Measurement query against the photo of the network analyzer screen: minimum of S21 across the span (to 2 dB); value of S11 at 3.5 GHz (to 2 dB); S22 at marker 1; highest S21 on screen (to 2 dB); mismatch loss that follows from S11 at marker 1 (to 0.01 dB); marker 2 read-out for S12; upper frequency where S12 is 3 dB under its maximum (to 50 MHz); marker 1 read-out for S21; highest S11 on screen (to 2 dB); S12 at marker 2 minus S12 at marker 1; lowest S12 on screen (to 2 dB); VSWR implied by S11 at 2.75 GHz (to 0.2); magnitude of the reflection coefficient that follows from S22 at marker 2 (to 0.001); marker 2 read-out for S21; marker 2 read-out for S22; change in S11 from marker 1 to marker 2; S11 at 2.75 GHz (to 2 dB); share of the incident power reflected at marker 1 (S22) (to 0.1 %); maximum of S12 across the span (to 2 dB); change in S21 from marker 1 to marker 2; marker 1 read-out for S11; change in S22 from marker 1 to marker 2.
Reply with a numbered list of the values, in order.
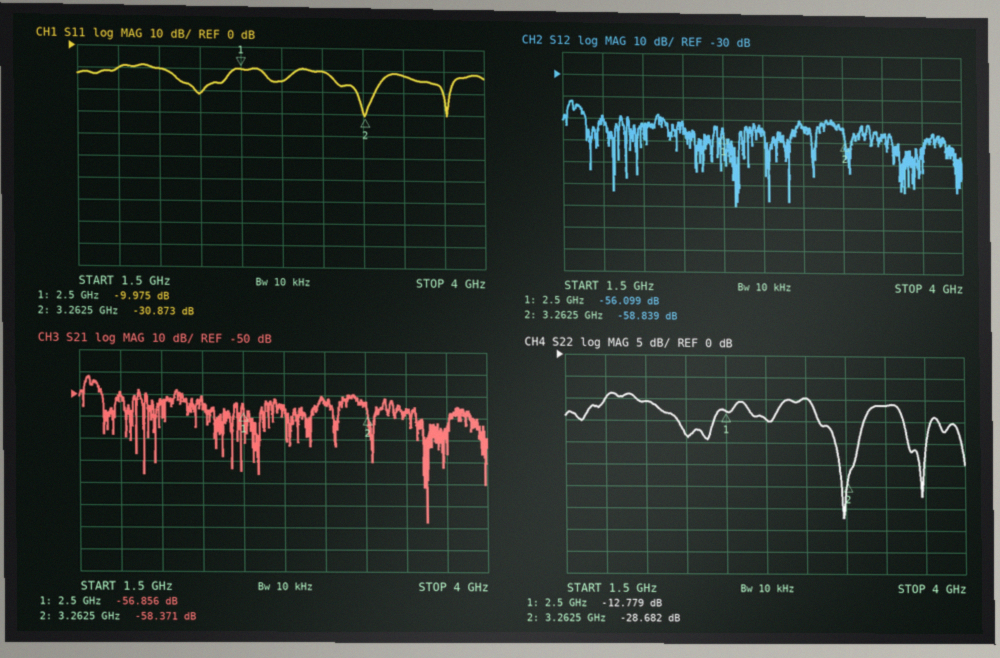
1. -108 dB
2. -12 dB
3. -12.779 dB
4. -42 dB
5. 0.46 dB
6. -58.839 dB
7. 1.55 GHz
8. -56.856 dB
9. -8 dB
10. -2.740 dB
11. -90 dB
12. 1.4
13. 0.037
14. -58.371 dB
15. -28.682 dB
16. -20.898 dB
17. -16 dB
18. 5.3 %
19. -42 dB
20. -1.515 dB
21. -9.975 dB
22. -15.903 dB
